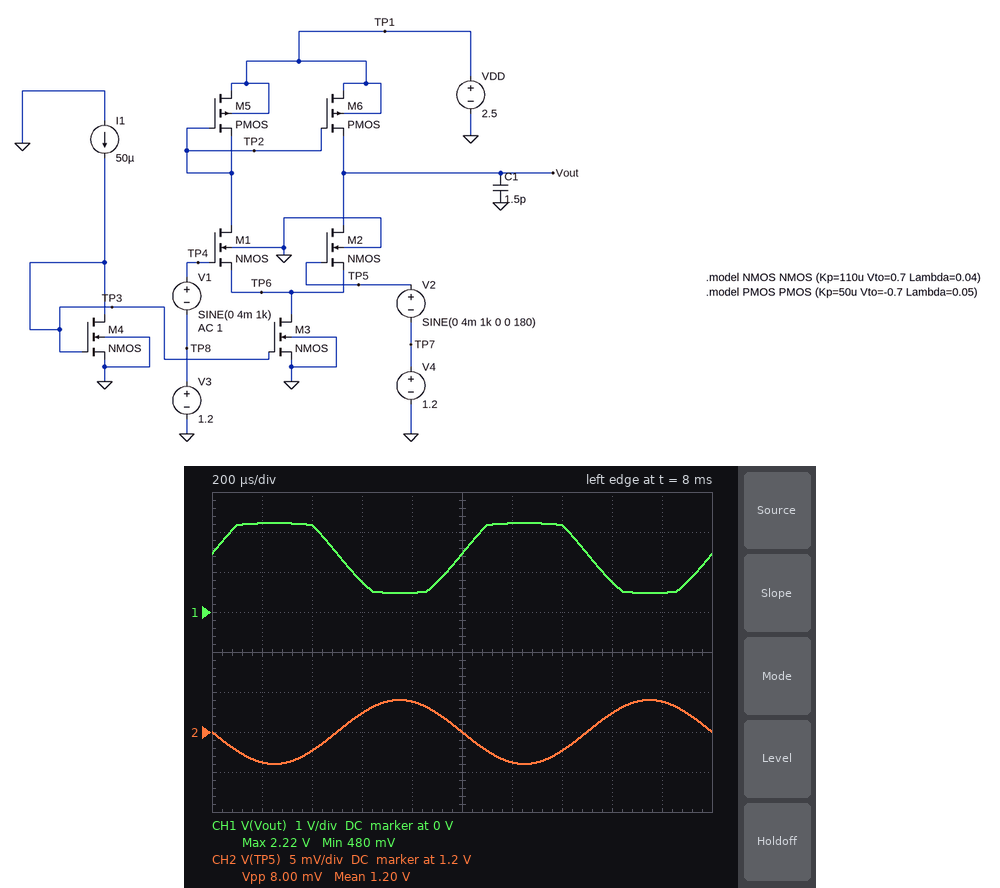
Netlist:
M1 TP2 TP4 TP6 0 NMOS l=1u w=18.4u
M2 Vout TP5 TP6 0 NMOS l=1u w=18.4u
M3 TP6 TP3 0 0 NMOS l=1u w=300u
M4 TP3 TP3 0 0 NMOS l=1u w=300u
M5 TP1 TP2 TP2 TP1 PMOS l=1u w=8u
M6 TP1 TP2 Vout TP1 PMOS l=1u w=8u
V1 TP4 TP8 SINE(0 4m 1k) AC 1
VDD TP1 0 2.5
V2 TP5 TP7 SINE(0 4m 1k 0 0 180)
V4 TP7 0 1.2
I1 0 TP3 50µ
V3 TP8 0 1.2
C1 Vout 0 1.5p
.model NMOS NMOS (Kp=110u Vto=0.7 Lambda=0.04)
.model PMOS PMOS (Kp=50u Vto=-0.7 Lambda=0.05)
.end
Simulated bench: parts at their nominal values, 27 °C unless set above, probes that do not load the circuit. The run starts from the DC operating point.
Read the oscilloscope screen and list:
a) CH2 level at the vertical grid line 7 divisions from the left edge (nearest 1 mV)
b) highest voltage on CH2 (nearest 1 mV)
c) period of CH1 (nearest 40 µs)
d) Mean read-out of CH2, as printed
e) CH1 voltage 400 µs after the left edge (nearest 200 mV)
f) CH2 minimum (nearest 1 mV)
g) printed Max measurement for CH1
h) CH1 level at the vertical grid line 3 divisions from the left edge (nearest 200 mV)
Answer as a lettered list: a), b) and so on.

a) 1.198 V
b) 1.204 V
c) 1.00 ms
d) 1.20 V
e) 2.2 V
f) 1.196 V
g) 2.22 V
h) 800 mV
